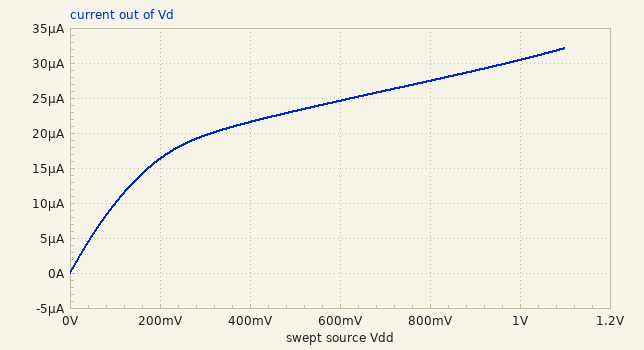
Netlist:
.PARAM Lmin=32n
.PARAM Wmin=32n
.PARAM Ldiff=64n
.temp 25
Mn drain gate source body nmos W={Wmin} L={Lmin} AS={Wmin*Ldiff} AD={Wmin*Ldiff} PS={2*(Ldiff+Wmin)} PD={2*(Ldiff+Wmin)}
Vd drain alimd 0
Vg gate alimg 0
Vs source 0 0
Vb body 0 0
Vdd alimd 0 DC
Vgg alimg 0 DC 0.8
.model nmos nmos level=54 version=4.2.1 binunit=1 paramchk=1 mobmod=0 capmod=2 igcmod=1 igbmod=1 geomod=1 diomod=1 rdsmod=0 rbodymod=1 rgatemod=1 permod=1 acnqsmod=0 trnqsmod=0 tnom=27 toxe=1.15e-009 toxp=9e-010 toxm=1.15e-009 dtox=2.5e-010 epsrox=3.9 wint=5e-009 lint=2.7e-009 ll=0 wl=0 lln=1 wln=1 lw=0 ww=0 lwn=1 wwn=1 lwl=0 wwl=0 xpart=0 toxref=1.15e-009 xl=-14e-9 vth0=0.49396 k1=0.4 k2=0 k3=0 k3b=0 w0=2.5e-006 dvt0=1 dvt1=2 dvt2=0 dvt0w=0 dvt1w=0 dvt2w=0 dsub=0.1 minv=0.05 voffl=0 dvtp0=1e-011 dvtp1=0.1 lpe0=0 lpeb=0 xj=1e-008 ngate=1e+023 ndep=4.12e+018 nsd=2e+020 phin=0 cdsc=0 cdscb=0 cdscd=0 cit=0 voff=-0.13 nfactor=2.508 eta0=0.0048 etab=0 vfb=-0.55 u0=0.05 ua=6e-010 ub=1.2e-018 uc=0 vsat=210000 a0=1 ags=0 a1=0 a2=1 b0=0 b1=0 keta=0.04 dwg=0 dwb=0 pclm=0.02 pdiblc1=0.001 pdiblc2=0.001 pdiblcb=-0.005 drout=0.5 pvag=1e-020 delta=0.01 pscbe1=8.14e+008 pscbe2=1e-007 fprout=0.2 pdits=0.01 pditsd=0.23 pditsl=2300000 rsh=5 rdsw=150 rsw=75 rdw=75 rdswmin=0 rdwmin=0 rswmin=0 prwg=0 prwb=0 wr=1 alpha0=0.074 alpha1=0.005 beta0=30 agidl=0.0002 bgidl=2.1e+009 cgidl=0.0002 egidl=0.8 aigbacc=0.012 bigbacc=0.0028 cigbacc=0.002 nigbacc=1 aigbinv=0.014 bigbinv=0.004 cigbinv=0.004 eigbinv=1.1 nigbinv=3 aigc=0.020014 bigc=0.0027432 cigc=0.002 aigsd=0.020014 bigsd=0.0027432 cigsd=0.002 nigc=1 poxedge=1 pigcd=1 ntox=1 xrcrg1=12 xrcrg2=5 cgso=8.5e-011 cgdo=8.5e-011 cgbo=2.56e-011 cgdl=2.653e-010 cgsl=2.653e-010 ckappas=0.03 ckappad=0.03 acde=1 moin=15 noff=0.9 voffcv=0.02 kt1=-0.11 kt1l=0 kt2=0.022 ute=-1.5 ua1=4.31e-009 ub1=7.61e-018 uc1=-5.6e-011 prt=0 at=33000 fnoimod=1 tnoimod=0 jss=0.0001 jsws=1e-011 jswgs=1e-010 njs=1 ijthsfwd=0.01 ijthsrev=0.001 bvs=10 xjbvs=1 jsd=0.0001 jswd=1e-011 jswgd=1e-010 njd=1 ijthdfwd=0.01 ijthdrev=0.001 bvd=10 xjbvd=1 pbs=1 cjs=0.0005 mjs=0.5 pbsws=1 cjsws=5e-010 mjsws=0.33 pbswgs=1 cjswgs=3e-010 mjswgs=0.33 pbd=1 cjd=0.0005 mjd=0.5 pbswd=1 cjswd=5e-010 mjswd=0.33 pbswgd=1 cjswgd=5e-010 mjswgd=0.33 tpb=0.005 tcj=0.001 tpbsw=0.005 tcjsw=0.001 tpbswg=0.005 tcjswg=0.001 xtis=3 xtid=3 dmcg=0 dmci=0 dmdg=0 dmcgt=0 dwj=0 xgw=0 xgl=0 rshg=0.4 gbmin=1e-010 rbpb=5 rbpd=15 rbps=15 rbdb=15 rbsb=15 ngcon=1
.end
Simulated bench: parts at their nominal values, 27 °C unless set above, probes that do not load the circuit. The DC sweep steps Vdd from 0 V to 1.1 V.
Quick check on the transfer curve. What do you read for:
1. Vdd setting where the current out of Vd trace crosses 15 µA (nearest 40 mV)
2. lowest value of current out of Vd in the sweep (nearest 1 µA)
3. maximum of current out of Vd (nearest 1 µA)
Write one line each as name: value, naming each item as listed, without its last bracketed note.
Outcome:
Vdd setting where the current out of Vd trace crosses 15 µA: 160 mV
lowest value of current out of Vd in the sweep: 0 A
maximum of current out of Vd: 32 µA
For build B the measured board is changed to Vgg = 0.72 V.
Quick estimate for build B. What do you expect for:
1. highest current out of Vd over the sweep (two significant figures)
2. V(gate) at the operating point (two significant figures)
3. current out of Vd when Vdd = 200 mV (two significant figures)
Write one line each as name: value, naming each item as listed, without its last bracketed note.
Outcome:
highest current out of Vd over the sweep: 27 µA
V(gate) at the operating point: 720 mV
current out of Vd when Vdd = 200 mV: 13 µA
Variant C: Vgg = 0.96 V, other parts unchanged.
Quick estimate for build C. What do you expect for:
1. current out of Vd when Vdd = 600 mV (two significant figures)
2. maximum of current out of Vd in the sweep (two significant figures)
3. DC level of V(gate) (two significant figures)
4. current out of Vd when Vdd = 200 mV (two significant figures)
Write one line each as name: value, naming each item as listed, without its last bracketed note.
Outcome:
current out of Vd when Vdd = 600 mV: 35 µA
maximum of current out of Vd in the sweep: 42 µA
DC level of V(gate): 960 mV
current out of Vd when Vdd = 200 mV: 21 µA
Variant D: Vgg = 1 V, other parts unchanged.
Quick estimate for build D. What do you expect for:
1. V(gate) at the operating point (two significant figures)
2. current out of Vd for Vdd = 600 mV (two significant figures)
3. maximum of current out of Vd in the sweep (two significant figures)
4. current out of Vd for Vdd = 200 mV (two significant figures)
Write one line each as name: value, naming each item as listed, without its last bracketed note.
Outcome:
V(gate) at the operating point: 1.0 V
current out of Vd for Vdd = 600 mV: 37 µA
maximum of current out of Vd in the sweep: 45 µA
current out of Vd for Vdd = 200 mV: 22 µA
